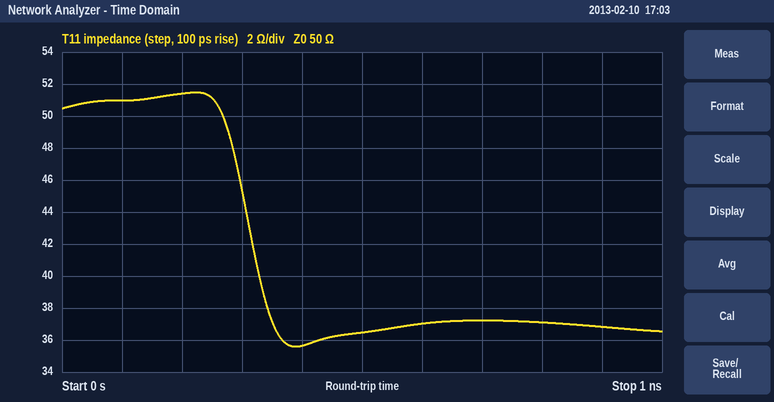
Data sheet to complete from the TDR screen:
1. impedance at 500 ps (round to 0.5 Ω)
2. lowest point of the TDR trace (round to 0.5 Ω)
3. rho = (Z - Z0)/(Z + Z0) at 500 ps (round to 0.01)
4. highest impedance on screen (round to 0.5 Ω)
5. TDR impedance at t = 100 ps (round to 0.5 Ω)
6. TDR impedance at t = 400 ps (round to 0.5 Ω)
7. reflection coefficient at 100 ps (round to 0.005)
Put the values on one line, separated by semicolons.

36.5 Ω; 35.5 Ω; -0.16; 51.5 Ω; 51.0 Ω; 35.5 Ω; +0.010
